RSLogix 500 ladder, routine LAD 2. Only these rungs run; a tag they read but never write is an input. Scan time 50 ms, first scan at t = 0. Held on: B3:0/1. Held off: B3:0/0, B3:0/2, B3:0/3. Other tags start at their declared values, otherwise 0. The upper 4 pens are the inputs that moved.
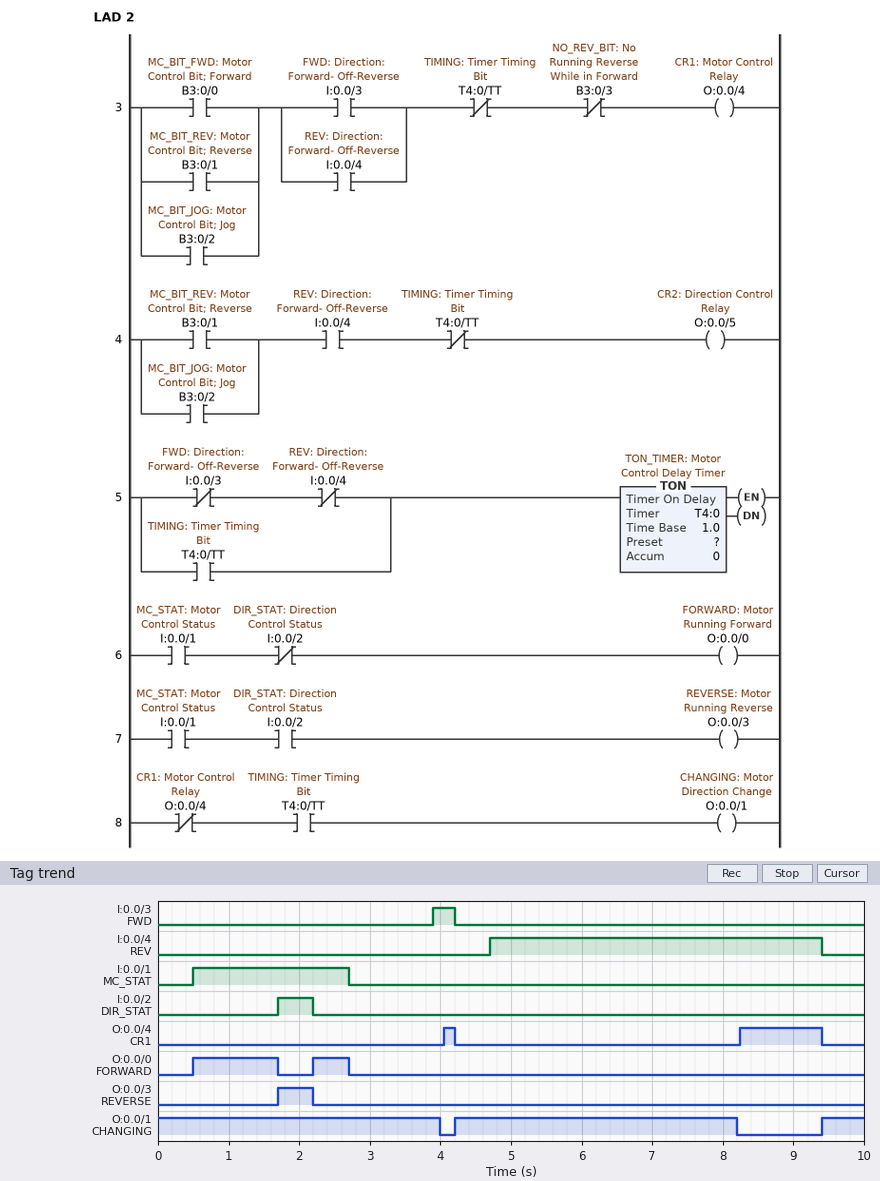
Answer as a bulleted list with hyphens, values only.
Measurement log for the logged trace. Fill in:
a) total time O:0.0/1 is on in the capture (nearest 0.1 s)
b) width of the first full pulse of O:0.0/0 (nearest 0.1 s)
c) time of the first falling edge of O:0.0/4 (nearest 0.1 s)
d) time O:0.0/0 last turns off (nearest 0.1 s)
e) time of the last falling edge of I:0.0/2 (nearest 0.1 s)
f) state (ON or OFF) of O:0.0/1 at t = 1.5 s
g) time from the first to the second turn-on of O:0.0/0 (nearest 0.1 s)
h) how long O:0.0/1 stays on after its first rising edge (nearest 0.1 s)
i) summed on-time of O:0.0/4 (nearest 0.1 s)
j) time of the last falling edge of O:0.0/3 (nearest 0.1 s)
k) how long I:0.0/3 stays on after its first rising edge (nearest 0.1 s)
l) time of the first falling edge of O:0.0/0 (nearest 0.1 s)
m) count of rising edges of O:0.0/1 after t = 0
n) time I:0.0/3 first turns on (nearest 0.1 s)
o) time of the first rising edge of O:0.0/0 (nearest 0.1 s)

- 8.6 s
- 1.2 s
- 4.2 s
- 2.7 s
- 2.2 s
- ON
- 1.7 s
- 4.0 s
- 1.3 s
- 2.2 s
- 0.3 s
- 1.7 s
- 2
- 3.9 s
- 0.5 s
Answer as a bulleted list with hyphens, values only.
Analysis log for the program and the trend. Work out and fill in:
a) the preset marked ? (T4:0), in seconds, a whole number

- 4 s
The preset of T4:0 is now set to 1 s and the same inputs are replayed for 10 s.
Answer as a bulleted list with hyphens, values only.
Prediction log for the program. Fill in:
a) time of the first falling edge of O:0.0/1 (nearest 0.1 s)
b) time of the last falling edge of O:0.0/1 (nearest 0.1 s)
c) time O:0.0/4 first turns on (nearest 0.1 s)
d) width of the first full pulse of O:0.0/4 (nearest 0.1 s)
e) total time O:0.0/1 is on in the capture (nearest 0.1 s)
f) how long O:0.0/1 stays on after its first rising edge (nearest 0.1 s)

- 1.0 s
- 5.2 s
- 3.9 s
- 0.3 s
- 2.6 s
- 1.0 s
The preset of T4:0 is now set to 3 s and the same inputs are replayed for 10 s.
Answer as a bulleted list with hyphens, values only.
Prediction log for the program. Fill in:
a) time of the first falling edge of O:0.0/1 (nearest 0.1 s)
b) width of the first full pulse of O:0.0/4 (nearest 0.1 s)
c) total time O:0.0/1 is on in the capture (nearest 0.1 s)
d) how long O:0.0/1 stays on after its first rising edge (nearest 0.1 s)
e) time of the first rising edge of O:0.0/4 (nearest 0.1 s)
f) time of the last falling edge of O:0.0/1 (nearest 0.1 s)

- 3.0 s
- 0.3 s
- 6.6 s
- 3.0 s
- 3.9 s
- 7.2 s
